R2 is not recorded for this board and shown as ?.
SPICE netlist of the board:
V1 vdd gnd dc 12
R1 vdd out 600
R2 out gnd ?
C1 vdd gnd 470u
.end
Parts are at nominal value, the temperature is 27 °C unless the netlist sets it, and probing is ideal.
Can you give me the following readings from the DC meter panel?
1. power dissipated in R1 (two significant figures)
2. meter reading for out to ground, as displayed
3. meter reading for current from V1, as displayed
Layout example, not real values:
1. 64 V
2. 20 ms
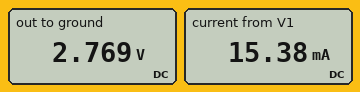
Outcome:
1. 140 mW
2. 2.769 V
3. 15.38 mA
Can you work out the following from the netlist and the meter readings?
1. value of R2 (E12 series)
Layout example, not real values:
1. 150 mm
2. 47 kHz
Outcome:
1. 180 Ω
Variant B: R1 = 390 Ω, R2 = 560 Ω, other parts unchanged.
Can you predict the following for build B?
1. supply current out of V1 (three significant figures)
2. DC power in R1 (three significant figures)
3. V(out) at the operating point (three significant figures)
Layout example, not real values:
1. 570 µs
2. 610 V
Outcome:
1. 12.6 mA
2. 62.2 mW
3. 7.07 V
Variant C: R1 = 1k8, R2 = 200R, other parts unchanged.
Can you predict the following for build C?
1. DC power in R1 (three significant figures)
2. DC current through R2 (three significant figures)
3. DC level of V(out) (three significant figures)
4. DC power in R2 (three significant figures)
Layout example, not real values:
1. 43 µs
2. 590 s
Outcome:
1. 64.8 mW
2. 6.00 mA
3. 1.20 V
4. 7.20 mW
